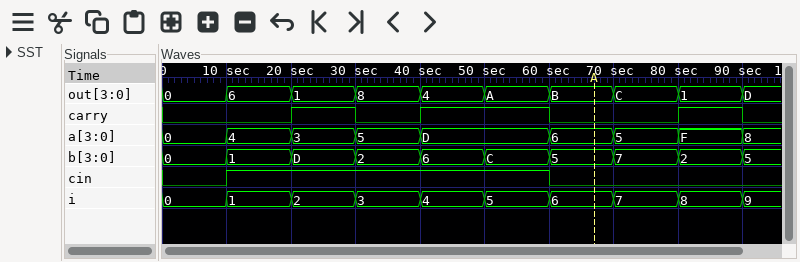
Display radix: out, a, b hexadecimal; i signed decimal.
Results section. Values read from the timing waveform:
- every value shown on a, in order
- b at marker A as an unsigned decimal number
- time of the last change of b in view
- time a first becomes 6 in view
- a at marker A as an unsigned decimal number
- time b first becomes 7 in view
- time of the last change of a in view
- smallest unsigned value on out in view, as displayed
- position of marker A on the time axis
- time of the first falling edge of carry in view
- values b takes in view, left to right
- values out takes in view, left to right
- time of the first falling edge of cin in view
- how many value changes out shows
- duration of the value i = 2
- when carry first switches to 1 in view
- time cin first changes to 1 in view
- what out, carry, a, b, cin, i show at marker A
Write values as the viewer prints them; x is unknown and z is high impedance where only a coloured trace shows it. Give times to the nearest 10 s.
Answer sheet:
0, 4, 3, 5, D, 6, 5, F, 8
5
90 s
60 s
6
70 s
90 s
0
70 s
30 s
0, 1, D, 2, 6, C, 5, 7, 2, 5
0, 6, 1, 8, 4, A, B, C, 1, D
60 s
9
10 s
20 s
10 s
out=B, carry=0, a=6, b=5, cin=0, i=6
